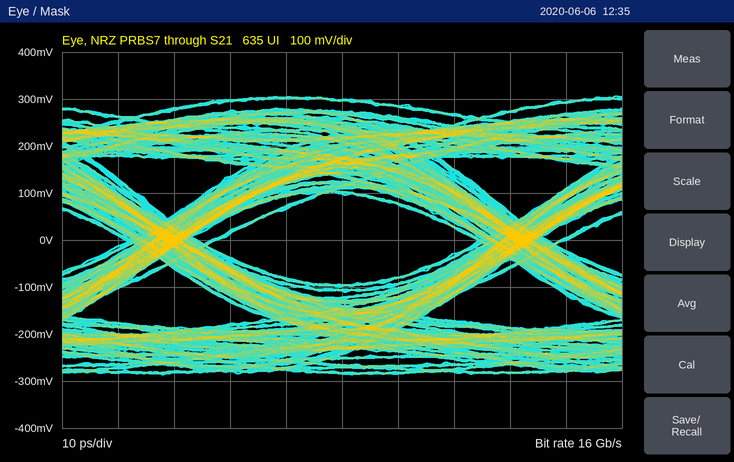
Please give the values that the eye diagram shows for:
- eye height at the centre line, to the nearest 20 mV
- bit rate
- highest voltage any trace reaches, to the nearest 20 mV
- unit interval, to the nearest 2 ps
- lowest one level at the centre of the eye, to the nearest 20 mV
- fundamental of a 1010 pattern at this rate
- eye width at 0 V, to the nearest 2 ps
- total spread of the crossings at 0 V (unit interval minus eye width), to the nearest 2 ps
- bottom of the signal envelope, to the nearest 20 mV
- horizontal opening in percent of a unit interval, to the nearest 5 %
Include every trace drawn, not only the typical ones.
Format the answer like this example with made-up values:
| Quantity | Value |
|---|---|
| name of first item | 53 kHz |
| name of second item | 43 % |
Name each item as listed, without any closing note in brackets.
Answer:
| Quantity | Value |
|---|---|
| eye height at the centre line, to the nearest 20 mV | 200 mV |
| bit rate | 16 Gb/s |
| highest voltage any trace reaches, to the nearest 20 mV | 300 mV |
| unit interval, to the nearest 2 ps | 62 ps |
| lowest one level at the centre of the eye, to the nearest 20 mV | 100 mV |
| fundamental of a 1010 pattern at this rate | 8 GHz |
| eye width at 0 V, to the nearest 2 ps | 46 ps |
| total spread of the crossings at 0 V (unit interval minus eye width), to the nearest 2 ps | 16 ps |
| bottom of the signal envelope, to the nearest 20 mV | -280 mV |
| horizontal opening in percent of a unit interval, to the nearest 5 % | 75 % |
